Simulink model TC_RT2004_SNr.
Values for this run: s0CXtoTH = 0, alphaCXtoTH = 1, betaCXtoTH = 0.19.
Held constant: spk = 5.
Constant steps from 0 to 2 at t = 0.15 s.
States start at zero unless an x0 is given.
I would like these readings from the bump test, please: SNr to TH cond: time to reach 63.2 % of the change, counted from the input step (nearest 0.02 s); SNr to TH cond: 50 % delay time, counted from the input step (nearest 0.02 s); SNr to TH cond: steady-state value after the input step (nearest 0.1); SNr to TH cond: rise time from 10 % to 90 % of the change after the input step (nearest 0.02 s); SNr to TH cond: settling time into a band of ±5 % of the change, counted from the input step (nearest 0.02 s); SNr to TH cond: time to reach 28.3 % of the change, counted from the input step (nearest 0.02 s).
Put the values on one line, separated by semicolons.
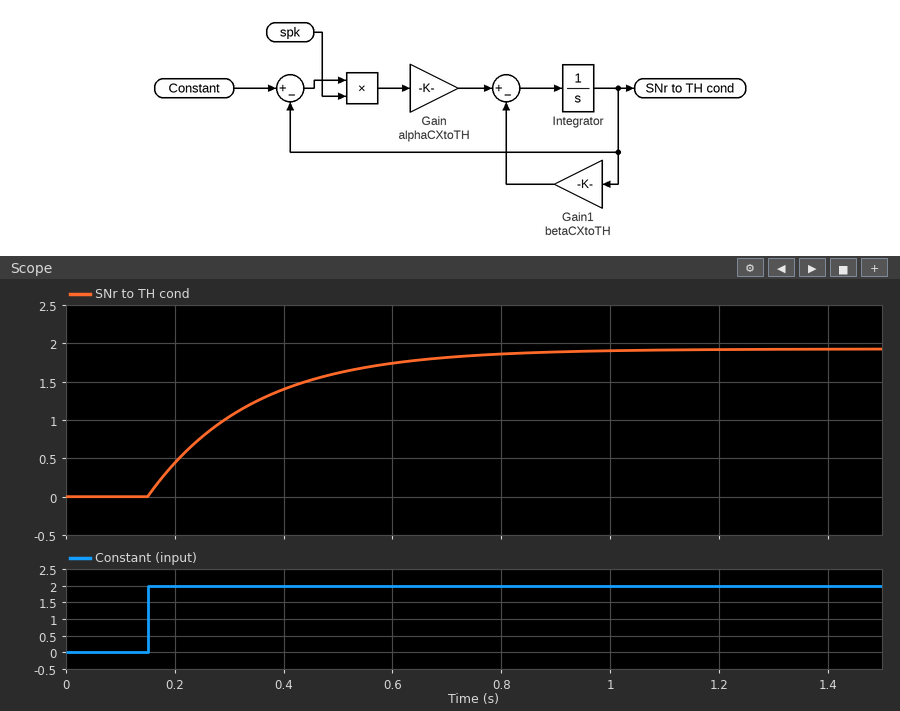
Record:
0.20 s; 0.14 s; 1.9; 0.42 s; 0.58 s; 0.06 s
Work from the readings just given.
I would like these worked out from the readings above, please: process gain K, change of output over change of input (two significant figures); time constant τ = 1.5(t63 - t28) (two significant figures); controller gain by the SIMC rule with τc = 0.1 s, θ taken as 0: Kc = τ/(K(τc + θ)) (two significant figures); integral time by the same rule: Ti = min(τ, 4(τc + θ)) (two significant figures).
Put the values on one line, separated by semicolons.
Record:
0.95; 0.21 s; 2.2; 0.21 s
